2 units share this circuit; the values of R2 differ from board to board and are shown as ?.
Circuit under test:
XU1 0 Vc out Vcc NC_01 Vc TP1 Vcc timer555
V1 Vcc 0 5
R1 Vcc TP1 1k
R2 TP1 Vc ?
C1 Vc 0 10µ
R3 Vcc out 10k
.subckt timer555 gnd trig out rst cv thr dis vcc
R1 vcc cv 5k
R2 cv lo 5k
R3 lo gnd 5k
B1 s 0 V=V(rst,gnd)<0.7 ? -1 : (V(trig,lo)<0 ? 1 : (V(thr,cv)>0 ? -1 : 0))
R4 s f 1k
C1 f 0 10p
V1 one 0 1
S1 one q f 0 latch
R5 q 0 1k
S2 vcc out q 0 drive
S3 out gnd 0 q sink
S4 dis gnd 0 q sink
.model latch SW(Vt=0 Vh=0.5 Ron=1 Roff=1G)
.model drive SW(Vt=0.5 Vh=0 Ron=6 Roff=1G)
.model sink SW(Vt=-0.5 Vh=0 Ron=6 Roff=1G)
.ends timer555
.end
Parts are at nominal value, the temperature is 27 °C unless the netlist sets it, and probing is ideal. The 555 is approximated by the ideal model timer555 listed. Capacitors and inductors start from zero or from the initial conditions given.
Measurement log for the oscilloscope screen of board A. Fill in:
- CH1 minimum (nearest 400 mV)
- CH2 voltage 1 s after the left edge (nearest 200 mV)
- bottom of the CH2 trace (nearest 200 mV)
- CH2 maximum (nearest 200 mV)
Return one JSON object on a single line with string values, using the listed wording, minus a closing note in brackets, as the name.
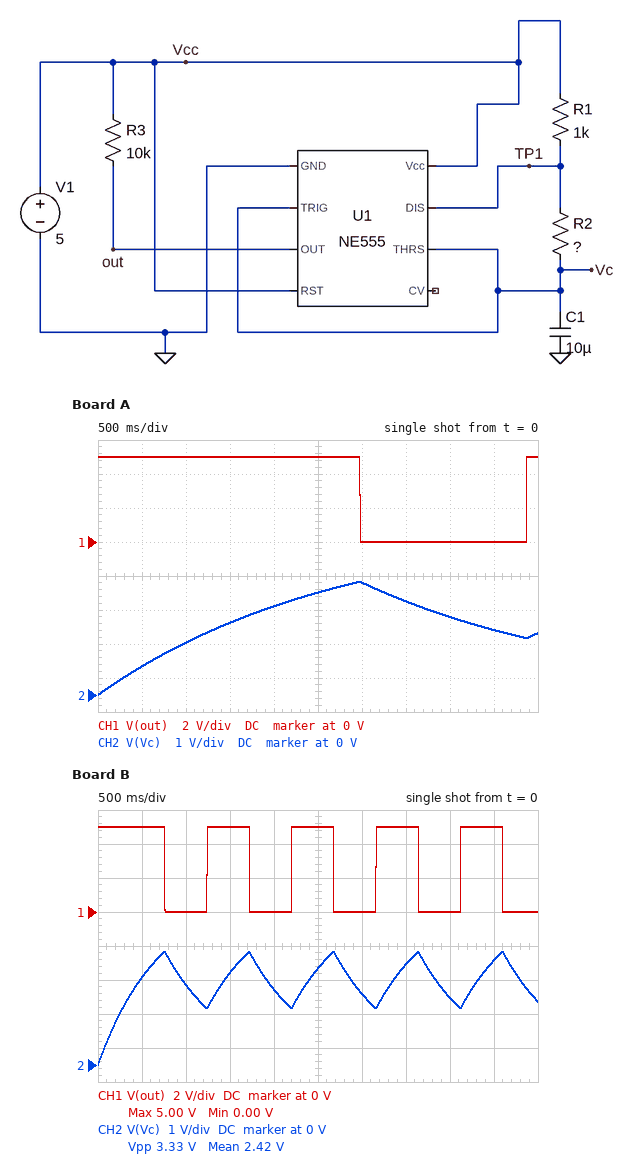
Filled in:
{"CH1 minimum": "0 V", "CH2 voltage 1 s after the left edge": "1.6 V", "bottom of the CH2 trace": "0 V", "CH2 maximum": "3.4 V"}
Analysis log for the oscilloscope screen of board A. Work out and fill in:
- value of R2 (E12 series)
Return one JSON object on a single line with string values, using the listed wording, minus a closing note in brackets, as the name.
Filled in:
{"value of R2": "270 kΩ"}
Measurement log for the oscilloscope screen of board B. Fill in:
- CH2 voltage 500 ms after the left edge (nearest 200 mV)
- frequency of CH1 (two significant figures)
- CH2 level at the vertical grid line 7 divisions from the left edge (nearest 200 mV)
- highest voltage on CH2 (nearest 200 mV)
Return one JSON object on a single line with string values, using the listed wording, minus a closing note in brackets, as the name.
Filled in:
{"CH2 voltage 500 ms after the left edge": "2.6 V", "frequency of CH1": "1.0 Hz", "CH2 level at the vertical grid line 7 divisions from the left edge": "3.0 V", "highest voltage on CH2": "3.4 V"}
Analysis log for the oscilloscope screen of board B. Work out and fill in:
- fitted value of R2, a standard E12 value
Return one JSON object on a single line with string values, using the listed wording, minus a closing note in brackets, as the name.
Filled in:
{"fitted value of R2, a standard E12 value": "68 kΩ"}
